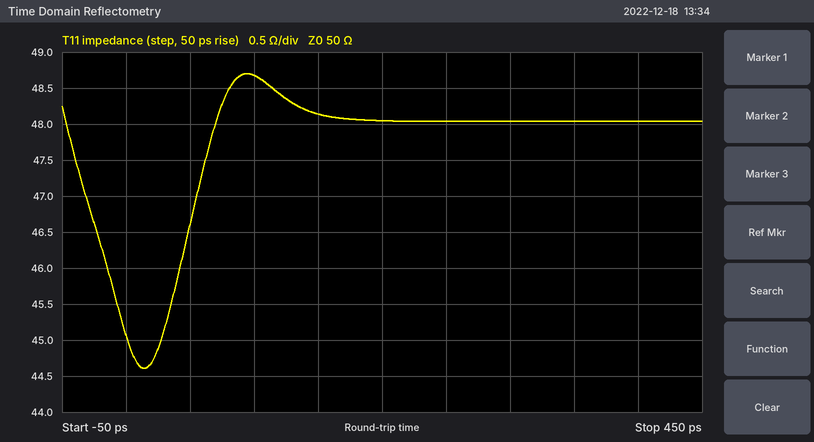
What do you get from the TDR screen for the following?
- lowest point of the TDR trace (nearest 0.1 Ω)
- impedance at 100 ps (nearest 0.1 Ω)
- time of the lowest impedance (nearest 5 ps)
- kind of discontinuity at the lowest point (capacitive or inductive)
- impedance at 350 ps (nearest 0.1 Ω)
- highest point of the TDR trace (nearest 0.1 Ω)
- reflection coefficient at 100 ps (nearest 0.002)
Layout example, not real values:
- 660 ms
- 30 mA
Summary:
- 44.6 Ω
- 48.7 Ω
- 15 ps
- capacitive
- 48.0 Ω
- 48.7 Ω
- -0.014
